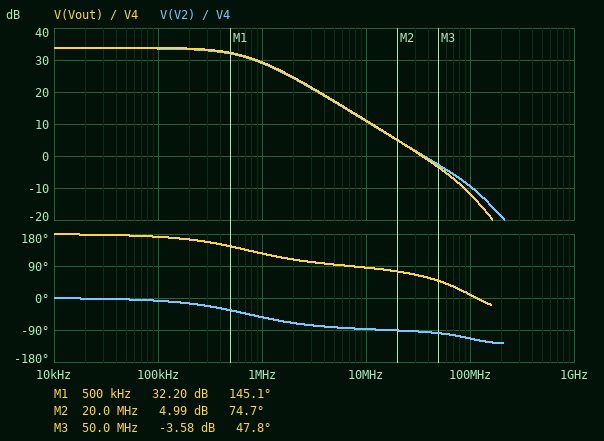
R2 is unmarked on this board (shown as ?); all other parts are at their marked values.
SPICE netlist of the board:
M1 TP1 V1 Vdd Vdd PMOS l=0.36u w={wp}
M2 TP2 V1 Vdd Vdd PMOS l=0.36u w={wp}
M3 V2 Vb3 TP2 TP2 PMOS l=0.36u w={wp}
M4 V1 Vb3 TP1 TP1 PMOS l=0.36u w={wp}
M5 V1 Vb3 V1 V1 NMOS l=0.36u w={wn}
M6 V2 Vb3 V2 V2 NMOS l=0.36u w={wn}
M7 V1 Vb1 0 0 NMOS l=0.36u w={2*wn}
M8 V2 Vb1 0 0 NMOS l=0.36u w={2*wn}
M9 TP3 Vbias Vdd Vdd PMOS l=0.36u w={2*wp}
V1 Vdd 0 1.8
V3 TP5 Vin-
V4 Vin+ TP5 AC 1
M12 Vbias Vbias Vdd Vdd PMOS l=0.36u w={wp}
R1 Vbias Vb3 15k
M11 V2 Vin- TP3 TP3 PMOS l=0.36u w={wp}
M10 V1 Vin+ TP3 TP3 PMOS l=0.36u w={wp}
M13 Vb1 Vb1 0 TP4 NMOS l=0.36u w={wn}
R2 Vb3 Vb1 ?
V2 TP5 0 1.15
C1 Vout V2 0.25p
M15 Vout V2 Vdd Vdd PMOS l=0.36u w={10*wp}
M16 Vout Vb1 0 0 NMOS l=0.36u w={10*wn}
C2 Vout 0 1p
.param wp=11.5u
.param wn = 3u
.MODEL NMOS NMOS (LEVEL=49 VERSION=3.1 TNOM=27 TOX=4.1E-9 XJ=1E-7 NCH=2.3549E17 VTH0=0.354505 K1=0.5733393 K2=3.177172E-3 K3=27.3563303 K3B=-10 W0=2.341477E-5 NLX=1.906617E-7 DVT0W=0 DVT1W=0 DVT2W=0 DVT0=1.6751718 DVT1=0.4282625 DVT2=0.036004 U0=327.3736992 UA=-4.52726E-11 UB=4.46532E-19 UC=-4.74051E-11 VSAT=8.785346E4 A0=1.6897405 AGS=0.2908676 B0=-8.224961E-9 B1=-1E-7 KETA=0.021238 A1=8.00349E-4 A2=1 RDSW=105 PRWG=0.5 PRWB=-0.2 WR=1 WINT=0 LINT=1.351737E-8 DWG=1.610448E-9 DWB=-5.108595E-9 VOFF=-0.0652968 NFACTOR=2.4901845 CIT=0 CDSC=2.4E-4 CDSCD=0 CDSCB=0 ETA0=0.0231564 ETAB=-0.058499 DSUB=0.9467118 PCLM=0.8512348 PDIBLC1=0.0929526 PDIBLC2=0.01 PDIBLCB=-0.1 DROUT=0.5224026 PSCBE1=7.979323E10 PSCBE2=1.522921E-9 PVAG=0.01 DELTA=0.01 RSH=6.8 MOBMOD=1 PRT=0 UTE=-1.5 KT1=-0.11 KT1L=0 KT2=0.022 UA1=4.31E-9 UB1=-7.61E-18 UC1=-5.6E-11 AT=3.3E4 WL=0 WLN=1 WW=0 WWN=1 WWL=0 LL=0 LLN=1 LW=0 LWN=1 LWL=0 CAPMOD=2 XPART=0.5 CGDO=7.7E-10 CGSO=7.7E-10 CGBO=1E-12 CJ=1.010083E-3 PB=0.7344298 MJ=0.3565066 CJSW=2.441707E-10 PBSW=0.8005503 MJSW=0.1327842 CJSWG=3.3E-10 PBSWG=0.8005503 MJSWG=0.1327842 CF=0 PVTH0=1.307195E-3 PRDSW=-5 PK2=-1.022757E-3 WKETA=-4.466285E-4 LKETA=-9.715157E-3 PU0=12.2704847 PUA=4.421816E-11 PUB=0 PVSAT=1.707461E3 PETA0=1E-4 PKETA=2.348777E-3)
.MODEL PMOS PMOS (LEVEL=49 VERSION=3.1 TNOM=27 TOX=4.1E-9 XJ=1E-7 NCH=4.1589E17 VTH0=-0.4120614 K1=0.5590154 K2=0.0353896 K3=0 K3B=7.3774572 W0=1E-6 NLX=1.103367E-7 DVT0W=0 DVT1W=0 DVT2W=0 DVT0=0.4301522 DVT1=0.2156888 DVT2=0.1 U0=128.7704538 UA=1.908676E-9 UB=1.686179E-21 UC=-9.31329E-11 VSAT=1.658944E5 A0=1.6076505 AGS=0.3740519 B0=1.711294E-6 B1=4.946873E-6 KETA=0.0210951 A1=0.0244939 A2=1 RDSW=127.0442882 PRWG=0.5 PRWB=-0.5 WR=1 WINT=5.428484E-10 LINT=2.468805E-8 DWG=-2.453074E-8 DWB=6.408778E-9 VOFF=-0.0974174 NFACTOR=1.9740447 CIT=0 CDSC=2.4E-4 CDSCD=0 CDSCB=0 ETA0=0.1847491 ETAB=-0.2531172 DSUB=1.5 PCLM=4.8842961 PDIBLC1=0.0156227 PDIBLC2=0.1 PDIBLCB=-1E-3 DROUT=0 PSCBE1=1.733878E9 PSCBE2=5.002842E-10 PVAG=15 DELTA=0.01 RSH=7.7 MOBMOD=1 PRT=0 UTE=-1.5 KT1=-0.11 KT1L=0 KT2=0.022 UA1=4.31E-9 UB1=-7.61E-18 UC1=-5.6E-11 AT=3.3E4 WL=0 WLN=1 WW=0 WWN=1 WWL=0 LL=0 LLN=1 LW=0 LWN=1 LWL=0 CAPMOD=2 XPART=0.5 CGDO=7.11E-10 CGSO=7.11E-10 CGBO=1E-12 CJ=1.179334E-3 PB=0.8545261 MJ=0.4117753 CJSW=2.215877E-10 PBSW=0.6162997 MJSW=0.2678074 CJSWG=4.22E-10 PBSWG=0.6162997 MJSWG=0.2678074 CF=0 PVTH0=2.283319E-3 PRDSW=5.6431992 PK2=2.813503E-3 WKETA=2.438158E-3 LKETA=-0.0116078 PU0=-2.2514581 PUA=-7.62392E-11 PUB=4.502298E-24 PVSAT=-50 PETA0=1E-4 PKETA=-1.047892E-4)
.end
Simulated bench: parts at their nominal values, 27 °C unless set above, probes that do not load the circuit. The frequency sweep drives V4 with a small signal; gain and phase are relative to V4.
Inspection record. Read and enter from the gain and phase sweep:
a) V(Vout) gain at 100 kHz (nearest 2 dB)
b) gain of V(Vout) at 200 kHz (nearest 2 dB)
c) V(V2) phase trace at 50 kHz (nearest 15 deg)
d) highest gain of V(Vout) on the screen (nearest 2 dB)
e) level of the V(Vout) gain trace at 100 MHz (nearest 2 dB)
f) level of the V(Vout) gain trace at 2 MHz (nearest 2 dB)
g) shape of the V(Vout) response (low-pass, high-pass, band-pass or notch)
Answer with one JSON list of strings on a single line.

["34 dB", "34 dB", "0 deg", "34 dB", "-12 dB", "24 dB", "low-pass"]
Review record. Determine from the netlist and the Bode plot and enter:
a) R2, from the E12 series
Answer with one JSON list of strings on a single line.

["10 kΩ"]
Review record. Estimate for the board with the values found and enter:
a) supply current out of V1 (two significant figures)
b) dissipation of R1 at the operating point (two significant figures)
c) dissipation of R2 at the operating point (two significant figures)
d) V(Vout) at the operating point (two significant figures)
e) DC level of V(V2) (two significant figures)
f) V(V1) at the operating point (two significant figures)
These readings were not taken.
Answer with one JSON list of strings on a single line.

["110 µA", "9.0 µW", "6.0 µW", "38 mV", "1.3 V", "1.3 V"]
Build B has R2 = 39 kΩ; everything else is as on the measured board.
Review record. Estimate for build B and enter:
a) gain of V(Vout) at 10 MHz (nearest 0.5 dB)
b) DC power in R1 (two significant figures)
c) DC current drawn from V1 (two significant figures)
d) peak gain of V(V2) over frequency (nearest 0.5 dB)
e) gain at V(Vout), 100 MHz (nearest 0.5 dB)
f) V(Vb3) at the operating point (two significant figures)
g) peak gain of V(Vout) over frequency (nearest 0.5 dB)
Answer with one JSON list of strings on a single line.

["-49.0 dB", "2.5 µW", "33 µA", "-14.5 dB", "-36.0 dB", "1.0 V", "-35.5 dB"]
